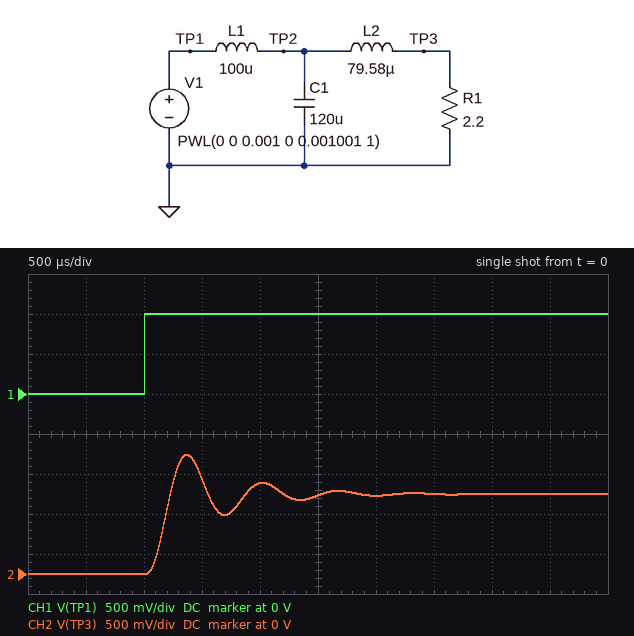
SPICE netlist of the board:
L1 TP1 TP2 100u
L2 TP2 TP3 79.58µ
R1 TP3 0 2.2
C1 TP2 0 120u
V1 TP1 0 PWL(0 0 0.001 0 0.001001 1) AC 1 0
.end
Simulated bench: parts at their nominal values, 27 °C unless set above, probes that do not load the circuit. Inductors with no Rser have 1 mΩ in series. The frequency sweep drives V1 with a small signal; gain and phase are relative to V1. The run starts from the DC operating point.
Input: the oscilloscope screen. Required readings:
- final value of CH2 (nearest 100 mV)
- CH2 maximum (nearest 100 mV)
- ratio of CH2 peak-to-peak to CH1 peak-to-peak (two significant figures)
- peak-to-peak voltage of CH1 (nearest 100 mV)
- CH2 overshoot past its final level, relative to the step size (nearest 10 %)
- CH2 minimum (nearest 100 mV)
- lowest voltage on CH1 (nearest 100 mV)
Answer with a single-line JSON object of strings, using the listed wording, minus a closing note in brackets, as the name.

{"final value of CH2": "1.0 V", "CH2 maximum": "1.5 V", "ratio of CH2 peak-to-peak to CH1 peak-to-peak": "1.5", "peak-to-peak voltage of CH1": "1.0 V", "CH2 overshoot past its final level, relative to the step size": "50 %", "CH2 minimum": "0 V", "lowest voltage on CH1": "0 V"}
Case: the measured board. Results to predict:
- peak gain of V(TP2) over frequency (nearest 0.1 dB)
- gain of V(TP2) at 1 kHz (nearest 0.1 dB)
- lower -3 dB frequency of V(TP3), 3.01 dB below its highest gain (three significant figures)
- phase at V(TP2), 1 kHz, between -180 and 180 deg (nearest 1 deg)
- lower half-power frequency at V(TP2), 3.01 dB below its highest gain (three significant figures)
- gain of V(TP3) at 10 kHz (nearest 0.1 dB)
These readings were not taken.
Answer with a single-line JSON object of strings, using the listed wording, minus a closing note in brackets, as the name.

{"peak gain of V(TP2) over frequency": "8.2 dB", "gain of V(TP2) at 1 kHz": "3.8 dB", "lower -3 dB frequency of V(TP3), 3.01 dB below its highest gain": "1.13 kHz", "phase at V(TP2), 1 kHz, between -180 and 180 deg": "-25 deg", "lower half-power frequency at V(TP2), 3.01 dB below its highest gain": "1.15 kHz", "gain of V(TP3) at 10 kHz": "-41.0 dB"}
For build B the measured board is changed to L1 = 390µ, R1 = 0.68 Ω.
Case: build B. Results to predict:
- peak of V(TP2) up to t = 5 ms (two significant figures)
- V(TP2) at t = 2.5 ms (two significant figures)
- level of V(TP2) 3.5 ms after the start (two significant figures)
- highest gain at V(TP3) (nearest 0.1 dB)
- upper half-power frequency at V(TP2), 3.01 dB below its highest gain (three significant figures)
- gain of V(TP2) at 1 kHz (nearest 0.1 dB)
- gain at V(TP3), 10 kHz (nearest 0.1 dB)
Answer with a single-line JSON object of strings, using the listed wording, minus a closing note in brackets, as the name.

{"peak of V(TP2) up to t = 5 ms": "1.0 V", "V(TP2) at t = 2.5 ms": "920 mV", "level of V(TP2) 3.5 ms after the start": "980 mV", "highest gain at V(TP3)": "0 dB", "upper half-power frequency at V(TP2), 3.01 dB below its highest gain": "274 Hz", "gain of V(TP2) at 1 kHz": "-7.9 dB", "gain at V(TP3), 10 kHz": "-62.5 dB"}
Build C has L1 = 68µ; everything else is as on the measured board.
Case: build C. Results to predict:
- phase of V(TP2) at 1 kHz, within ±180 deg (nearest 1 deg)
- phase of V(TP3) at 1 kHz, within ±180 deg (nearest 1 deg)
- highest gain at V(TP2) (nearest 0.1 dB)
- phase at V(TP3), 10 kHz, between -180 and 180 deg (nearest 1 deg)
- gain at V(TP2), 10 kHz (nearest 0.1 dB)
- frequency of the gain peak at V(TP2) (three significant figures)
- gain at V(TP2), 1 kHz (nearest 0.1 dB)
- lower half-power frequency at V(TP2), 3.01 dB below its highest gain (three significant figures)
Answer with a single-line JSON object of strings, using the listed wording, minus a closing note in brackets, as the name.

{"phase of V(TP2) at 1 kHz, within ±180 deg": "-14 deg", "phase of V(TP3) at 1 kHz, within ±180 deg": "-27 deg", "highest gain at V(TP2)": "10.2 dB", "phase at V(TP3), 10 kHz, between -180 and 180 deg": "114 deg", "gain at V(TP2), 10 kHz": "-29.7 dB", "frequency of the gain peak at V(TP2)": "1.84 kHz", "gain at V(TP2), 1 kHz": "2.6 dB", "lower half-power frequency at V(TP2), 3.01 dB below its highest gain": "1.52 kHz"}
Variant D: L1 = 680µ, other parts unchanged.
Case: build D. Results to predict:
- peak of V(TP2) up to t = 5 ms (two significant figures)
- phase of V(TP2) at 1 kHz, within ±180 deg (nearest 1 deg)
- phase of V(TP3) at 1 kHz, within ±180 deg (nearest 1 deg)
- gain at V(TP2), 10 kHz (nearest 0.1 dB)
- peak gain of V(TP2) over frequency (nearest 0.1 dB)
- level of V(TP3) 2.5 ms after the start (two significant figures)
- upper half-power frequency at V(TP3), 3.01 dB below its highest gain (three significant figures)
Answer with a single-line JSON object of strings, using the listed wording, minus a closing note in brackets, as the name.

{"peak of V(TP2) up to t = 5 ms": "1.1 V", "phase of V(TP2) at 1 kHz, within ±180 deg": "-134 deg", "phase of V(TP3) at 1 kHz, within ±180 deg": "-147 deg", "gain at V(TP2), 10 kHz": "-49.9 dB", "peak gain of V(TP2) over frequency": "0.5 dB", "level of V(TP3) 2.5 ms after the start": "1.0 V", "upper half-power frequency at V(TP3), 3.01 dB below its highest gain": "681 Hz"}
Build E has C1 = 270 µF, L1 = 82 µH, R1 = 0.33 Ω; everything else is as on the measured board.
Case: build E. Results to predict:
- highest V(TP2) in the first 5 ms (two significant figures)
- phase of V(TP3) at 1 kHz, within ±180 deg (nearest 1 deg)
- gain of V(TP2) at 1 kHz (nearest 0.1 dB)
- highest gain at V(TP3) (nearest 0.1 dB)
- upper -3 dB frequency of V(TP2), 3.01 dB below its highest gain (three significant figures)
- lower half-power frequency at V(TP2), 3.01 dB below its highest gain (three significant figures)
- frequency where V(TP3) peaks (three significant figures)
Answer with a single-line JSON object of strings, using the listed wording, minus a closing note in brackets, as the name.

{"highest V(TP2) in the first 5 ms": "1.2 V", "phase of V(TP3) at 1 kHz, within ±180 deg": "-86 deg", "gain of V(TP2) at 1 kHz": "0.3 dB", "highest gain at V(TP3)": "0.5 dB", "upper -3 dB frequency of V(TP2), 3.01 dB below its highest gain": "1.62 kHz", "lower half-power frequency at V(TP2), 3.01 dB below its highest gain": "1.29 kHz", "frequency where V(TP3) peaks": "1.45 kHz"}
